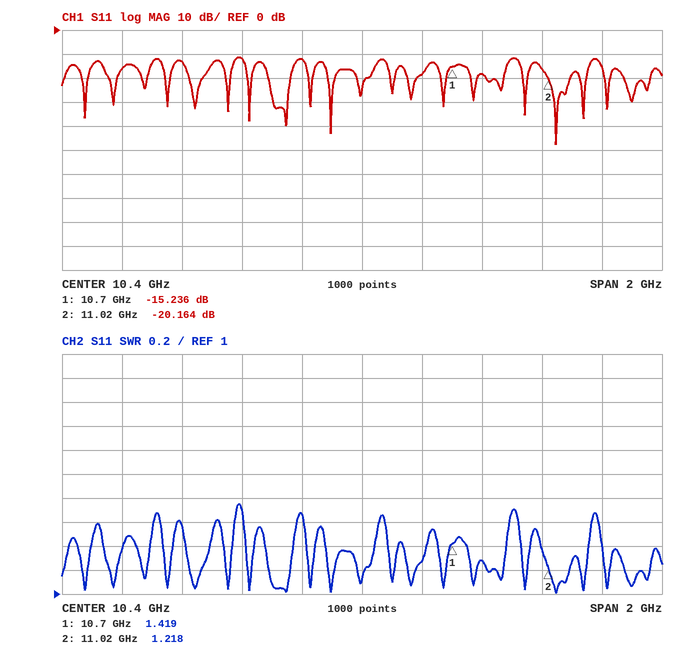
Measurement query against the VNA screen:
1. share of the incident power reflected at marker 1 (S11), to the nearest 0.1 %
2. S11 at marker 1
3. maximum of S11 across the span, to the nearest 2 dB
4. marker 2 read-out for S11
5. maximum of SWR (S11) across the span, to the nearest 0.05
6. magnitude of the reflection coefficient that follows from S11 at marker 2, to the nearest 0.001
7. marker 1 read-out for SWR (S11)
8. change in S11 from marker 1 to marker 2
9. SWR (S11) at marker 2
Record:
3.0 %
-15.236 dB
-12 dB
-20.164 dB
1.75
0.098
1.419
-4.928 dB
1.218
